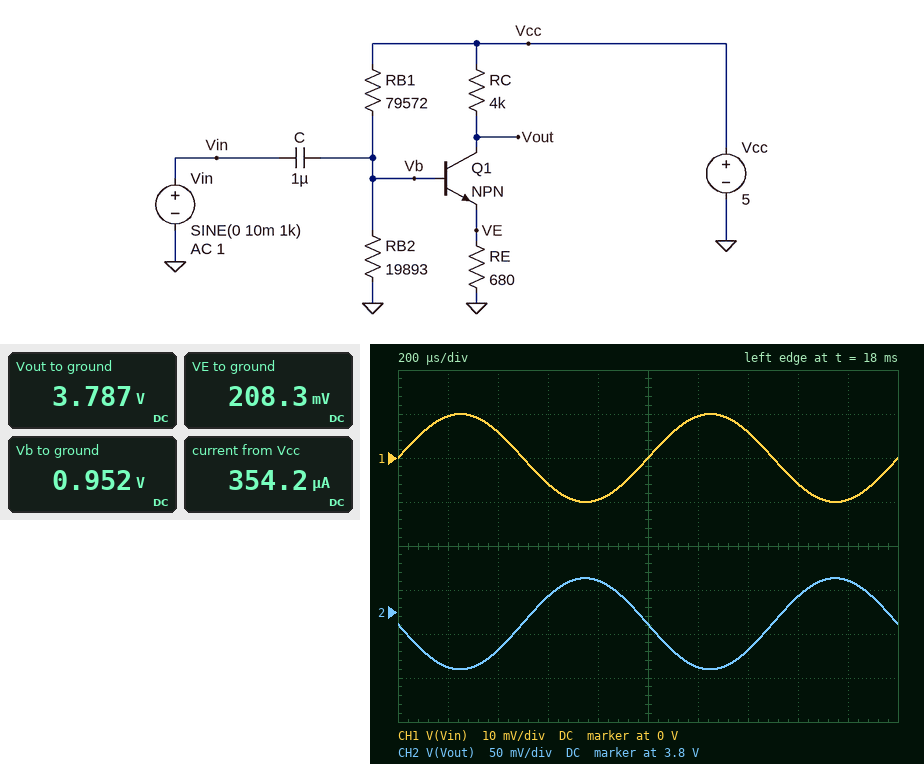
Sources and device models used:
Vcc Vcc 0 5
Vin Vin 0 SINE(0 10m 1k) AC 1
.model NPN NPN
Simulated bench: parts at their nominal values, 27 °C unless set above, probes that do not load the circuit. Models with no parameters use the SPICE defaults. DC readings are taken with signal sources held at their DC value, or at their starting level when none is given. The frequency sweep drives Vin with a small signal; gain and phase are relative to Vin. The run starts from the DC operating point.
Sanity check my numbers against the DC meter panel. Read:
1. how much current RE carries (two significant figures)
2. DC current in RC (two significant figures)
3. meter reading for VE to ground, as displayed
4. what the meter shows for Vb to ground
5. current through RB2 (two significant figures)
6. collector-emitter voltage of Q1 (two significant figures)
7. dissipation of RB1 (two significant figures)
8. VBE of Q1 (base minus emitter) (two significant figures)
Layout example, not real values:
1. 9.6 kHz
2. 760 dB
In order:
1. 310 µA
2. 300 µA
3. 208.3 mV
4. 0.952 V
5. 48 µA
6. 3.6 V
7. 210 µW
8. 740 mV
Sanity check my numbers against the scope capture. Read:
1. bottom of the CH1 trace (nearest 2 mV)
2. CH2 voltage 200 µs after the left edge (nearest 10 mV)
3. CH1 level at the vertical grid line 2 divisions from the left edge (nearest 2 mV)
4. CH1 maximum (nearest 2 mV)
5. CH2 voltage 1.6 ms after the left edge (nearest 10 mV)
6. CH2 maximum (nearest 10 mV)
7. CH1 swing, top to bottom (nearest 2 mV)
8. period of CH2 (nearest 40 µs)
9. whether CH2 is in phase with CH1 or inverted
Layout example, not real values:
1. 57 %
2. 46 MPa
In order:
1. -10 mV
2. 3.74 V
3. 6 mV
4. 10 mV
5. 3.82 V
6. 3.84 V
7. 20 mV
8. 1.00 ms
9. inverted
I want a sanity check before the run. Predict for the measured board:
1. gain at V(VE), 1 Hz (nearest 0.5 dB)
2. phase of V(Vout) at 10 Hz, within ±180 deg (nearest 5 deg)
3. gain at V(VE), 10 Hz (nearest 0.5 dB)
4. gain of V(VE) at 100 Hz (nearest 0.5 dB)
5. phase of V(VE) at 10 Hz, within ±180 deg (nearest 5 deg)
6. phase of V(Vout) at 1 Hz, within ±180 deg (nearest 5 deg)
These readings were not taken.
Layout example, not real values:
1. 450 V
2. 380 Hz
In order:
1. -22.5 dB
2. -130 deg
3. -5.0 dB
4. -1.0 dB
5. 50 deg
6. -95 deg
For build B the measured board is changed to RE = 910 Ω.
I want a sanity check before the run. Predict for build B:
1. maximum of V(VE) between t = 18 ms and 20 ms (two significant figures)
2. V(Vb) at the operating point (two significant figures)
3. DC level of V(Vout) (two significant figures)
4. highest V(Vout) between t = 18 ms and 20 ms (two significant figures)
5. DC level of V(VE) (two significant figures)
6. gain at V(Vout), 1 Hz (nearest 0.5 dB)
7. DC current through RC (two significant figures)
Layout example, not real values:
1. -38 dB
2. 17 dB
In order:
1. 230 mV
2. 960 mV
3. 4.0 V
4. 4.1 V
5. 220 mV
6. -9.5 dB
7. 240 µA
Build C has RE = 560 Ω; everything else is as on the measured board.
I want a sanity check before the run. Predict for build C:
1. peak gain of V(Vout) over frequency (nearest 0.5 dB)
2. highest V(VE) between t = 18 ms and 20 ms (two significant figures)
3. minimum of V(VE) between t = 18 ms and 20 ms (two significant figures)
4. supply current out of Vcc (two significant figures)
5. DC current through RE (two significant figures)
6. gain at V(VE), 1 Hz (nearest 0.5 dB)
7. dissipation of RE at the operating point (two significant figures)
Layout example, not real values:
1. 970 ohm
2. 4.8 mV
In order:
1. 16.0 dB
2. 210 mV
3. 190 mV
4. 400 µA
5. 350 µA
6. -23.0 dB
7. 70 µW
